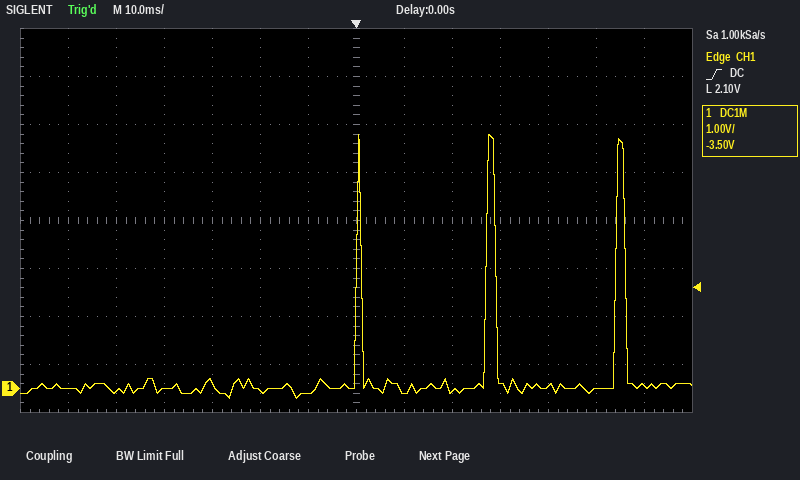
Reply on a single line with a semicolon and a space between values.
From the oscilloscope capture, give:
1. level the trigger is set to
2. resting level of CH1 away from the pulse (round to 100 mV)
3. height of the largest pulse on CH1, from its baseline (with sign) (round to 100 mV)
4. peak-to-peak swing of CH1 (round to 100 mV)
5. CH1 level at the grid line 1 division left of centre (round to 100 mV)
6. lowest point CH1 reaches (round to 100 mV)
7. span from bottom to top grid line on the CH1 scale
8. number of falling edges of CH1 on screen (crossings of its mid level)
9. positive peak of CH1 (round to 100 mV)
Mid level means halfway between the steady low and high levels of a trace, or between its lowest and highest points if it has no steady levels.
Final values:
2.10 V; 0.0 V; +5.3 V; 5.5 V; -100 mV; -200 mV; 8 V; 3; 5.3 V
